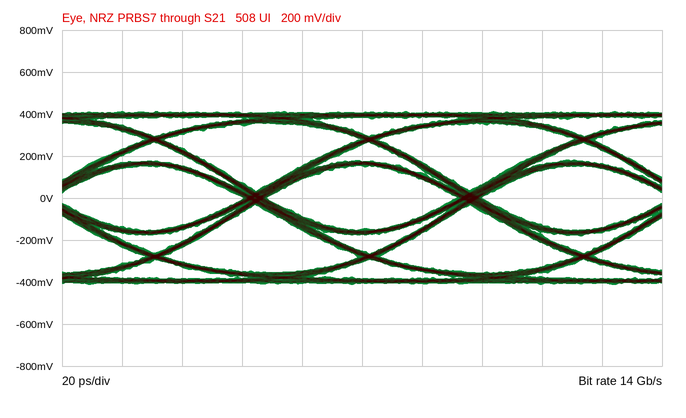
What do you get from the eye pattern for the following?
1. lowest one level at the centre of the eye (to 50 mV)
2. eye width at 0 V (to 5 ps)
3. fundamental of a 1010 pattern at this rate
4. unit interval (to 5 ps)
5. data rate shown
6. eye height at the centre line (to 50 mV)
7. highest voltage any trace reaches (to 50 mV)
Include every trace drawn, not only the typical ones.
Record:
150 mV
65 ps
7 GHz
70 ps
14 Gb/s
300 mV
400 mV
